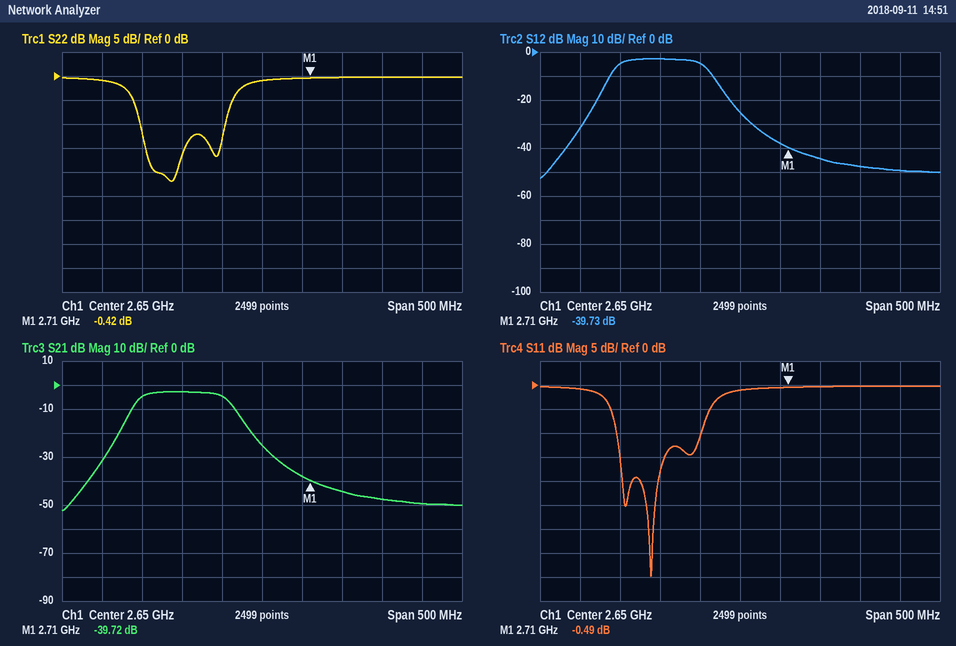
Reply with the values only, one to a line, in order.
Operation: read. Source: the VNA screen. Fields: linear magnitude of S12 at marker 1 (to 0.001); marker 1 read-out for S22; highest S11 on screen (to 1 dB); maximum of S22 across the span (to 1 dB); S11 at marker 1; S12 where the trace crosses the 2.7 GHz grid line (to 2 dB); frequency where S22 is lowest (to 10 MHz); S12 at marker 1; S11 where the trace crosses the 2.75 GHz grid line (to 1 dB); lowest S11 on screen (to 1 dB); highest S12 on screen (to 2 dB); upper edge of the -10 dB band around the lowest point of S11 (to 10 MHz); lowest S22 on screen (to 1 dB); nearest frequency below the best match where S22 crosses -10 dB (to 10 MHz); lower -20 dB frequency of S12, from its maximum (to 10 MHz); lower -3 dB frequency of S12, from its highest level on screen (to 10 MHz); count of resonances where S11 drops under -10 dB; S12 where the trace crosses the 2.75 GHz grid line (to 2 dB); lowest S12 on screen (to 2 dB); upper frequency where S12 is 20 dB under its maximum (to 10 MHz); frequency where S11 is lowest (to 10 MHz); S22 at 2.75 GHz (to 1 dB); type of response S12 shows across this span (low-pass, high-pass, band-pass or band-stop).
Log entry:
0.010
-0.42 dB
0 dB
0 dB
-0.49 dB
-38 dB
2.54 GHz
-39.73 dB
0 dB
-40 dB
-2 dB
2.60 GHz
-22 dB
2.50 GHz
2.47 GHz
2.50 GHz
2
-44 dB
-52 dB
2.64 GHz
2.54 GHz
0 dB
band-pass
